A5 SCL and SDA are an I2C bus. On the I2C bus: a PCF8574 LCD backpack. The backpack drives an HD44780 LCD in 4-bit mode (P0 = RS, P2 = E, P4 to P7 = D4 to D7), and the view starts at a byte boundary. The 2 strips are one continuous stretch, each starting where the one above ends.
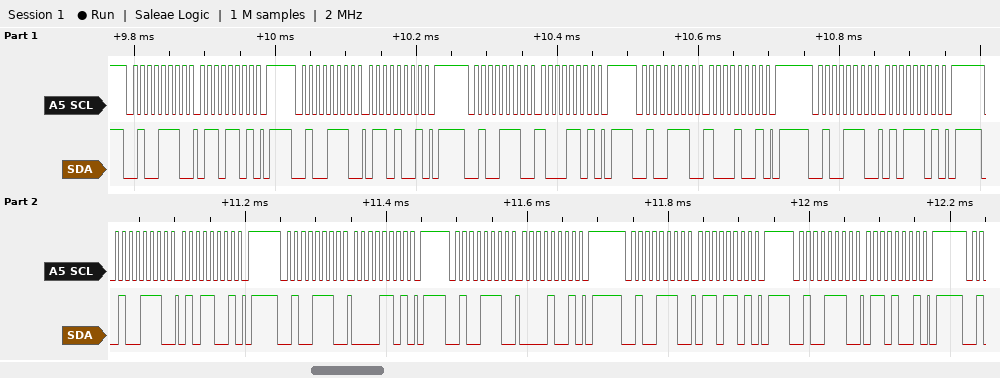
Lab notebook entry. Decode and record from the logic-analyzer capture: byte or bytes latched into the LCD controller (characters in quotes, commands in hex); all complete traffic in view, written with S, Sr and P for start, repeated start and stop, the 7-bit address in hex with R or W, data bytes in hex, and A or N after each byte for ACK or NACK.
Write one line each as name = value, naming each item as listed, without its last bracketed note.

byte or bytes latched into the LCD controller = 'h' 'P'
all complete traffic in view, written with S, Sr and P for start, repeated start and stop, the 7-bit address in hex with R or W, data bytes in hex, and A or N after each byte for ACK or NACK = S 27W A 6D A P S 27W A 69 A P S 27W A 8D A P S 27W A 89 A P S 27W A 5D A P S 27W A 59 A P S 27W A 0D A P S 27W A 09 A P S 27W A 6D A P S 27W A 69 A P
